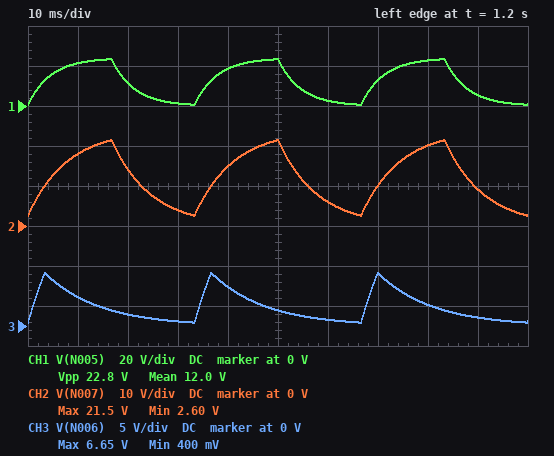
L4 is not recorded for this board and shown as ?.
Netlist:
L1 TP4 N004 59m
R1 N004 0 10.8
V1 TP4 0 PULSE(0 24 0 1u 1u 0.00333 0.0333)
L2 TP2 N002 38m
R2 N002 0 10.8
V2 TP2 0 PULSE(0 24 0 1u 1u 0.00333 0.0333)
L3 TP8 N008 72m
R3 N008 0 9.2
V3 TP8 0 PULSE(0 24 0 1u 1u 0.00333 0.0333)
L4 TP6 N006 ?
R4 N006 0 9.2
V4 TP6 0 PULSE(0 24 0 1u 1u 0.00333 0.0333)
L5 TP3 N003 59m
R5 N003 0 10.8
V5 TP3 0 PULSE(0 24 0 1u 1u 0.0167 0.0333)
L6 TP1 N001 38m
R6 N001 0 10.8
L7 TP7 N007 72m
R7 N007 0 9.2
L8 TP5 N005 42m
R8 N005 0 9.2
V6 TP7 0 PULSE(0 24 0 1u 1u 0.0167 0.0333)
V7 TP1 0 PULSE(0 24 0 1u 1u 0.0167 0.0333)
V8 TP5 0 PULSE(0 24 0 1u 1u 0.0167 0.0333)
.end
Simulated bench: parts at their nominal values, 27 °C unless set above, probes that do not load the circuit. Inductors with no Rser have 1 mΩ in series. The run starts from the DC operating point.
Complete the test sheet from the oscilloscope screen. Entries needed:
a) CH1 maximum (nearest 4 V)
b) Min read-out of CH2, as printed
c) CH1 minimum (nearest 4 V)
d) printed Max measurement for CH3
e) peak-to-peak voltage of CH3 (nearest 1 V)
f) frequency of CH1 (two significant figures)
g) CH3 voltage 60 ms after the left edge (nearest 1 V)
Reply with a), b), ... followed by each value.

a) 24 V
b) 2.60 V
c) 0 V
d) 6.65 V
e) 6 V
f) 30 Hz
g) 1 V
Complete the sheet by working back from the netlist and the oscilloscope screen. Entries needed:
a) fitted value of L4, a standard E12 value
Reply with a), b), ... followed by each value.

a) 100 mH
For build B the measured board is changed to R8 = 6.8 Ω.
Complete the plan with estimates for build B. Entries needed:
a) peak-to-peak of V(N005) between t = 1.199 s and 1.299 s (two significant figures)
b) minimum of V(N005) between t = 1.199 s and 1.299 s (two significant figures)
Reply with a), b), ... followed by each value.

a) 21 V
b) 1.5 V
